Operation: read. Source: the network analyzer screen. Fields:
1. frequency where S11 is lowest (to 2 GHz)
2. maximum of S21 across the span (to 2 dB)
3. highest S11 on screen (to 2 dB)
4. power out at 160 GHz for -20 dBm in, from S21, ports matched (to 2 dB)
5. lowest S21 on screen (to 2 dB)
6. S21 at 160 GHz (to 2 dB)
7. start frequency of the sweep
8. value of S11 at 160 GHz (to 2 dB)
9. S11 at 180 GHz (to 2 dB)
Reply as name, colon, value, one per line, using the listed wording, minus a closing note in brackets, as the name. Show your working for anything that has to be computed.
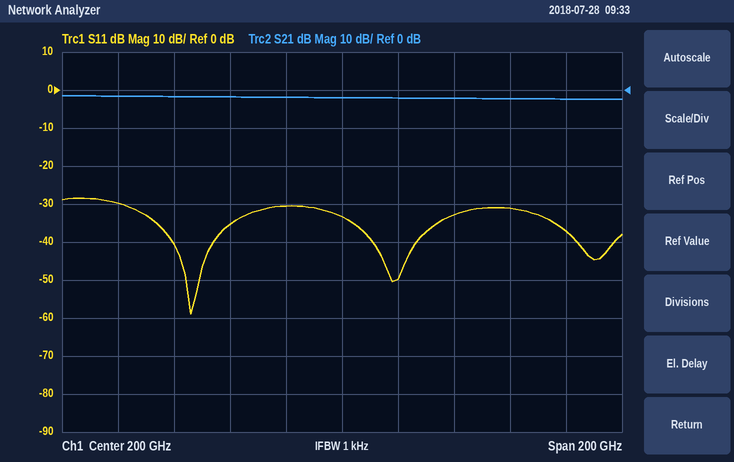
frequency where S11 is lowest: 146 GHz
maximum of S21 across the span: -2 dB
highest S11 on screen: -28 dB
power out at 160 GHz for -20 dBm in, from S21, ports matched: -20 dBm + (-2 dB) = -22 dBm
lowest S21 on screen: -2 dB
S21 at 160 GHz: -2 dB
start frequency of the sweep: 100 GHz
value of S11 at 160 GHz: -36 dB
S11 at 180 GHz: -30 dB
